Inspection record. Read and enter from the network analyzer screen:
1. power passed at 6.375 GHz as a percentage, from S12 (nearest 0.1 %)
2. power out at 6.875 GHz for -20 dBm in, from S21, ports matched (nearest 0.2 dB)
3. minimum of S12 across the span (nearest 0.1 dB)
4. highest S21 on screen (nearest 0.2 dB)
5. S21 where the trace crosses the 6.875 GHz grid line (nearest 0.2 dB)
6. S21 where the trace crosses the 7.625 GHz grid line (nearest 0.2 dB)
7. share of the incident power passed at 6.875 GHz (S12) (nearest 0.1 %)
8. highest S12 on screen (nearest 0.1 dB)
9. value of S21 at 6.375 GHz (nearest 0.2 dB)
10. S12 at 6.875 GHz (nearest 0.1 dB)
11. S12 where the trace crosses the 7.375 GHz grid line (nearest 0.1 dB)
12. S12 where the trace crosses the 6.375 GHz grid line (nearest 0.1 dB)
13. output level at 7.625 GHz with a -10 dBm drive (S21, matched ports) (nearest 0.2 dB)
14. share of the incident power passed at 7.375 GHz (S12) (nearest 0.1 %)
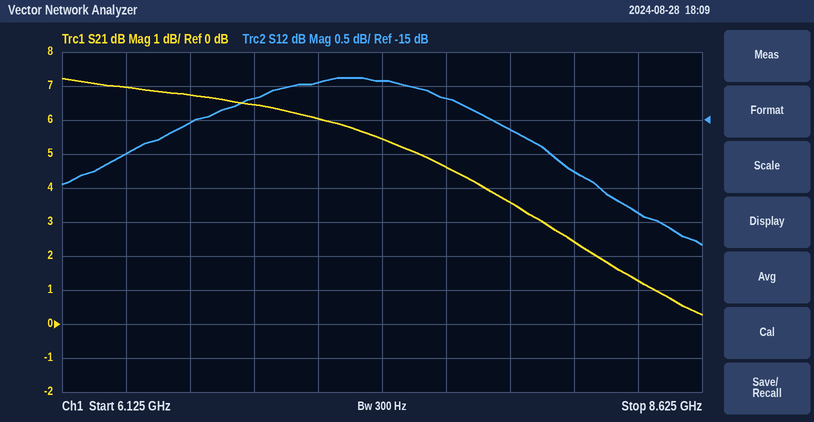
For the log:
2.8 %
-13.6 dBm
-16.8 dB
7.2 dB
6.4 dB
4.6 dB
3.4 %
-14.4 dB
7.0 dB
-14.7 dB
-14.4 dB
-15.5 dB
-5.4 dBm
3.6 %
